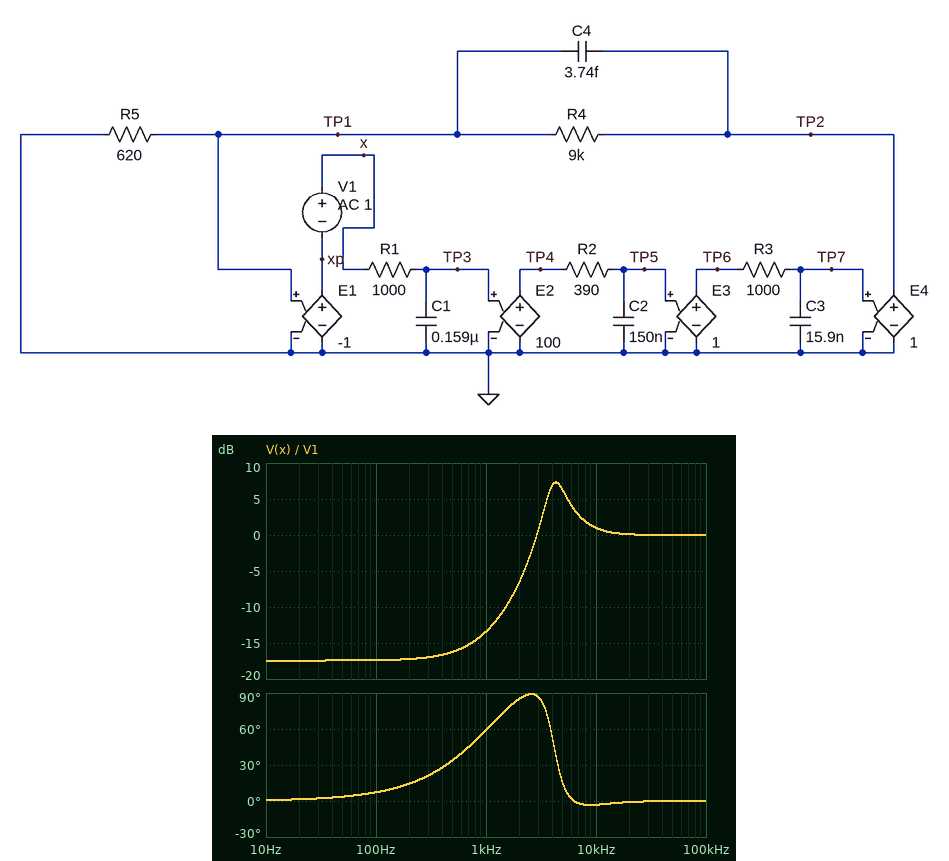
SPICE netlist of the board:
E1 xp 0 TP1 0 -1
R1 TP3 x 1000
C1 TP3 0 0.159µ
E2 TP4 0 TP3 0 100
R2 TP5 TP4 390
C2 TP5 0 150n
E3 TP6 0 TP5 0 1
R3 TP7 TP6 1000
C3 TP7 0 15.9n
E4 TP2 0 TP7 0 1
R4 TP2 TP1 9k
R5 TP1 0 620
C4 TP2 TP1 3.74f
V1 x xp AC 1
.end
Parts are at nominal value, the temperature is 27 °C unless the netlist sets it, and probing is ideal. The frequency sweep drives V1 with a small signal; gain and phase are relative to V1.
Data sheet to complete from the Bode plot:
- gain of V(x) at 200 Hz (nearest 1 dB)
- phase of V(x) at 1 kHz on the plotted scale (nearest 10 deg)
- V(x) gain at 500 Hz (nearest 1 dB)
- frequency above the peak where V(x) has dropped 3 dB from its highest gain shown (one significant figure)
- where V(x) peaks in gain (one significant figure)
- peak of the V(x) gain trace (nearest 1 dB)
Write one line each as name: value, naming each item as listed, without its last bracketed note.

gain of V(x) at 200 Hz: -17 dB
phase of V(x) at 1 kHz on the plotted scale: 60 deg
V(x) gain at 500 Hz: -16 dB
frequency above the peak where V(x) has dropped 3 dB from its highest gain shown: 6 kHz
where V(x) peaks in gain: 4 kHz
peak of the V(x) gain trace: 7 dB
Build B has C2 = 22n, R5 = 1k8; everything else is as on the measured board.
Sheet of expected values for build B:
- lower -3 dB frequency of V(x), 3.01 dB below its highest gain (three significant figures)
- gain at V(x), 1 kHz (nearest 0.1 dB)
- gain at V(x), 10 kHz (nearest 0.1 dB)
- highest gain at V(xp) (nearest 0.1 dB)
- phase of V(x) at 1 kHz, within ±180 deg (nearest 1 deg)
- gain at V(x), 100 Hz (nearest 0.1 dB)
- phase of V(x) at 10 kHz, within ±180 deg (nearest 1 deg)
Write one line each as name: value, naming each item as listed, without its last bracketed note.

lower -3 dB frequency of V(x), 3.01 dB below its highest gain: 9.88 kHz
gain at V(x), 1 kHz: -21.8 dB
gain at V(x), 10 kHz: 8.0 dB
highest gain at V(xp): 9.3 dB
phase of V(x) at 1 kHz, within ±180 deg: 50 deg
gain at V(x), 100 Hz: -24.9 dB
phase of V(x) at 10 kHz, within ±180 deg: 84 deg
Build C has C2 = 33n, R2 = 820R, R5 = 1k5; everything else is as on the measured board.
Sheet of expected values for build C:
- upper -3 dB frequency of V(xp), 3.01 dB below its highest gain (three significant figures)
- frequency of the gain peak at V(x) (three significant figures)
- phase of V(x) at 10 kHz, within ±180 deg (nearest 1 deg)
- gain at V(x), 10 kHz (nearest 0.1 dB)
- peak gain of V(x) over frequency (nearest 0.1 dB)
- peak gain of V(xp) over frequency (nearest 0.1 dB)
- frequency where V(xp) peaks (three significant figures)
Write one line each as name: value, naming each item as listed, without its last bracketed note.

upper -3 dB frequency of V(xp), 3.01 dB below its highest gain: 8.04 kHz
frequency of the gain peak at V(x): 7.59 kHz
phase of V(x) at 10 kHz, within ±180 deg: -9 deg
gain at V(x), 10 kHz: 6.0 dB
peak gain of V(x) over frequency: 15.8 dB
peak gain of V(xp) over frequency: 15.1 dB
frequency where V(xp) peaks: 7.51 kHz
